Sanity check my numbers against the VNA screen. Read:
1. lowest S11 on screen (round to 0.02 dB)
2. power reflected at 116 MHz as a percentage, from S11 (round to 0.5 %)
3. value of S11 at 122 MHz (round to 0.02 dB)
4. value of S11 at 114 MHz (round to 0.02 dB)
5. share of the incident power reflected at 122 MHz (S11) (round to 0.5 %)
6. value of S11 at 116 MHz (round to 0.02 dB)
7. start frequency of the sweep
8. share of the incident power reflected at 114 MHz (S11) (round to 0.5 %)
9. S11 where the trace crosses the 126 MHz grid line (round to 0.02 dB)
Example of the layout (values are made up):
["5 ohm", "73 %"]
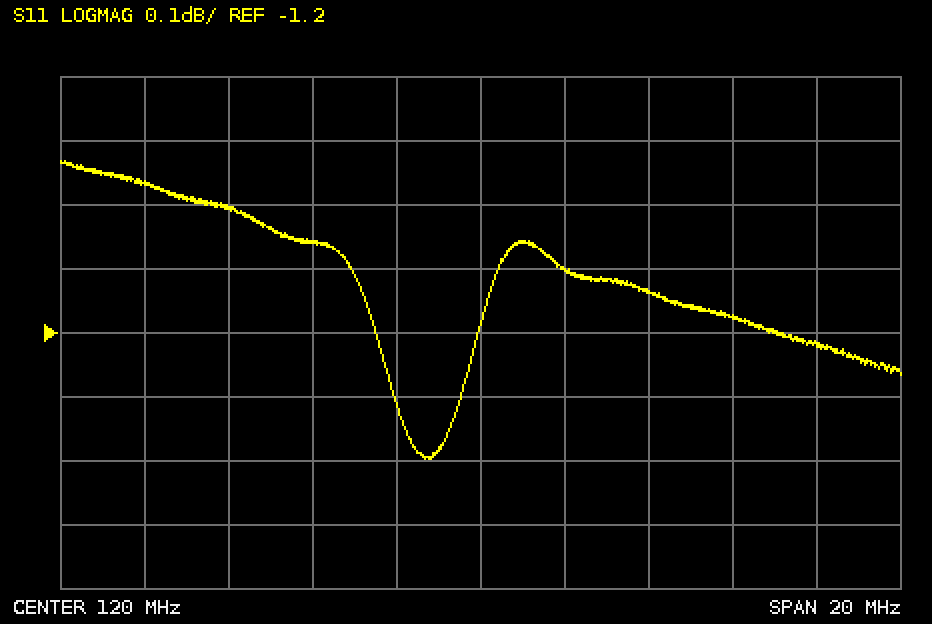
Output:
["-1.40 dB", "78.5 %", "-1.10 dB", "-1.00 dB", "77.5 %", "-1.06 dB", "110 MHz", "79.5 %", "-1.18 dB"]
